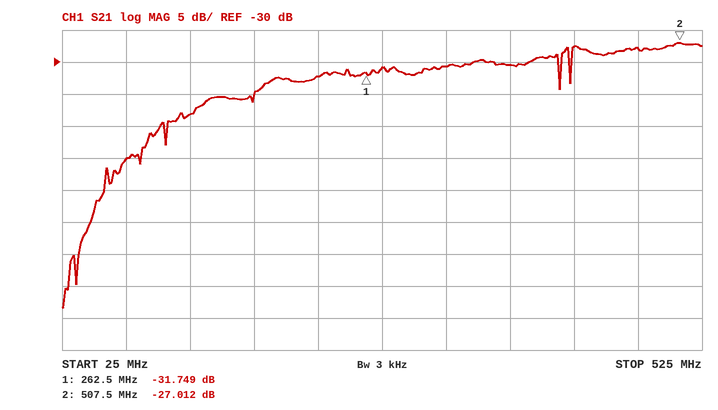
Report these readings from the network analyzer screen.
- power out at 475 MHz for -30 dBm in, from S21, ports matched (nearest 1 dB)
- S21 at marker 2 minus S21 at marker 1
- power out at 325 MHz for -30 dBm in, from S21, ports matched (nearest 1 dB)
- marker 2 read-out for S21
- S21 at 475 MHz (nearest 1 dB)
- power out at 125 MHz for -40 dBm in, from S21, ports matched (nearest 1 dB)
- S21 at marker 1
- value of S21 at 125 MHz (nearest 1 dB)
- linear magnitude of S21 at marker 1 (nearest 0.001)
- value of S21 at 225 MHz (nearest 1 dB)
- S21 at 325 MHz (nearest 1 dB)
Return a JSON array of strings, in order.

["-58 dBm", "4.737 dB", "-61 dBm", "-27.012 dB", "-28 dB", "-78 dBm", "-31.749 dB", "-38 dB", "0.026", "-32 dB", "-31 dB"]
